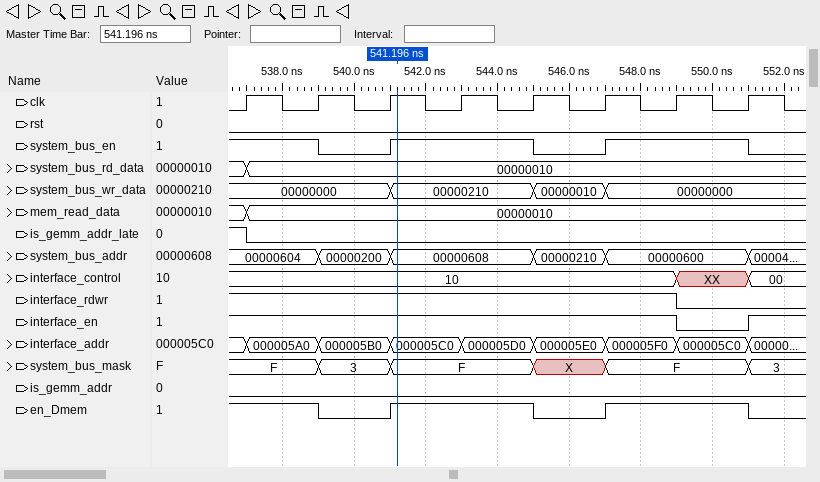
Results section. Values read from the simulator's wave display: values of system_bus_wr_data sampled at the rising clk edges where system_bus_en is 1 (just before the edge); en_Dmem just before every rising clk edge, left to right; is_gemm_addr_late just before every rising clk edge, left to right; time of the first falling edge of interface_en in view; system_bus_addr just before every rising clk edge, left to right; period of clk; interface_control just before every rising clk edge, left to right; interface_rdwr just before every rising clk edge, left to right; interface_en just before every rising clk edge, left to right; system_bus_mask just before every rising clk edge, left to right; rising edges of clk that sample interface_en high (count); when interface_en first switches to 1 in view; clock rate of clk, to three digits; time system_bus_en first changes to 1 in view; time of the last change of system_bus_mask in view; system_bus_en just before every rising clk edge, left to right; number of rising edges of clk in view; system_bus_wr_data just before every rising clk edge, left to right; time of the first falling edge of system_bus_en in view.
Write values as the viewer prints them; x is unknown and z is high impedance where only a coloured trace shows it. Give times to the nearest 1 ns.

00000000, 00000000, 00000210, 00000210, 00000000, 00000000
1 1 0 1 1 0 1 1
1 0 0 0 0 0 0 0
549 ns
00000604, 00000604, 00000200, 00000608, 00000608, 00000210, 00000600, 00000600
2 ns
10, 10, 10, 10, 10, 10, 10, XX
1 1 1 1 1 1 1 0
1 1 1 1 1 1 1 0
F, F, 3, F, F, X, F, F
7
551 ns
500 MHz
541 ns
551 ns
1 1 0 1 1 0 1 1
8
00000000, 00000000, 00000000, 00000210, 00000210, 00000010, 00000000, 00000000
539 ns
